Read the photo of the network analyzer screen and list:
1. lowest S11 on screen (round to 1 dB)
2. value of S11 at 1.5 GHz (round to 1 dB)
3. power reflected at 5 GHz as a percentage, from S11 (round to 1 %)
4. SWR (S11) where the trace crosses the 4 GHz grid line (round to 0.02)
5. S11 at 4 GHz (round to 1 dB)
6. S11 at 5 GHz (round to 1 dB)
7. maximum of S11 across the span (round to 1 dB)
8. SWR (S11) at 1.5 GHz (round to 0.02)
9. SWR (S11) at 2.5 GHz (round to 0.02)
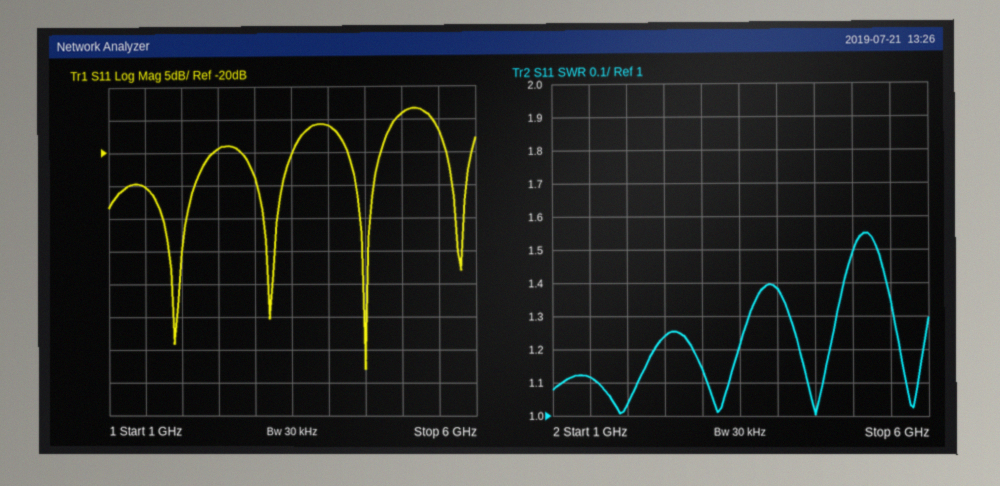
-53 dB
-25 dB
4 %
1.38
-16 dB
-14 dB
-13 dB
1.12
1.24
